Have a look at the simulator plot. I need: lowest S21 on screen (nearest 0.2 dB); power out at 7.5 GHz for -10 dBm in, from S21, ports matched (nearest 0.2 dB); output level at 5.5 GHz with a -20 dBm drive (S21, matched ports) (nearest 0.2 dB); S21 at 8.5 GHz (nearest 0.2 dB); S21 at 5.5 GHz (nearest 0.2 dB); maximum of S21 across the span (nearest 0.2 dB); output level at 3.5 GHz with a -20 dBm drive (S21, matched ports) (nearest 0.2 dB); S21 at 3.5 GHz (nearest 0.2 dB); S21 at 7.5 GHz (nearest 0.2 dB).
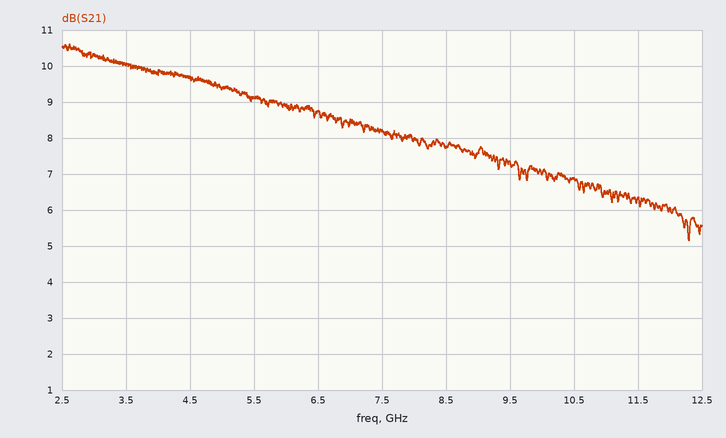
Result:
5.2 dB
-1.8 dBm
-10.8 dBm
7.8 dB
9.2 dB
10.6 dB
-10.0 dBm
10.0 dB
8.2 dB
